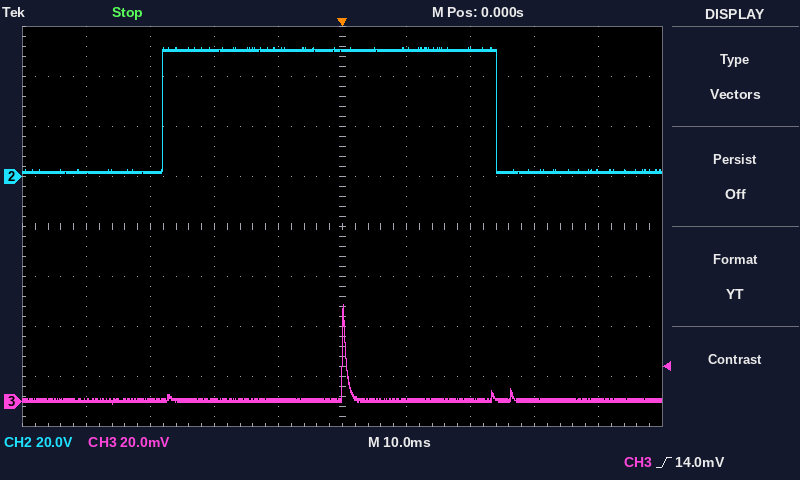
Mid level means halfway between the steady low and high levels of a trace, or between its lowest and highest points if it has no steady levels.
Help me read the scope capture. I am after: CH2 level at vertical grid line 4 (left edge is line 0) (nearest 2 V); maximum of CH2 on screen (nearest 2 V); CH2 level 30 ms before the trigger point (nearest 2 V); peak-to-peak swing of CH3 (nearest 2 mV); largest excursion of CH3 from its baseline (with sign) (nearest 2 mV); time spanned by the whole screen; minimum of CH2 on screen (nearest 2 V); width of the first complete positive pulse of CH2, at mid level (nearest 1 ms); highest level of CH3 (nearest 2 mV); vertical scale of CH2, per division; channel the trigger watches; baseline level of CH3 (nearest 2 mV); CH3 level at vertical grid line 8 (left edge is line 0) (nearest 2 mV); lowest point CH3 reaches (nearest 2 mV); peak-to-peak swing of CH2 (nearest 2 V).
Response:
50 V
52 V
2 V
40 mV
+38 mV
100 ms
2 V
52 ms
38 mV
20 V
CH3
0 mV
0 mV
-2 mV
50 V
